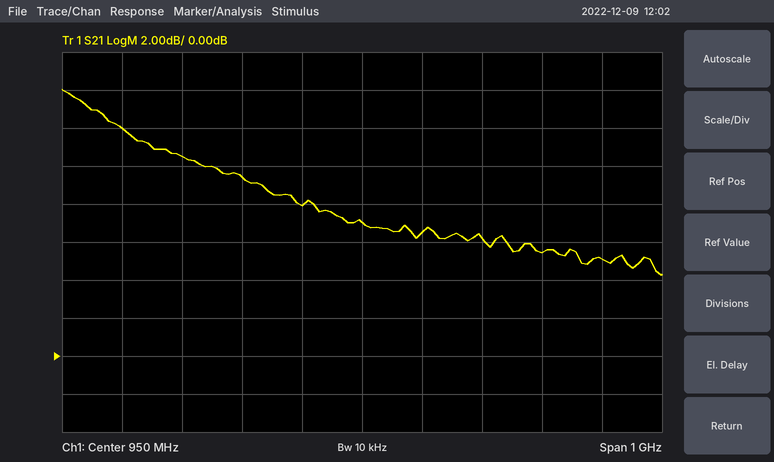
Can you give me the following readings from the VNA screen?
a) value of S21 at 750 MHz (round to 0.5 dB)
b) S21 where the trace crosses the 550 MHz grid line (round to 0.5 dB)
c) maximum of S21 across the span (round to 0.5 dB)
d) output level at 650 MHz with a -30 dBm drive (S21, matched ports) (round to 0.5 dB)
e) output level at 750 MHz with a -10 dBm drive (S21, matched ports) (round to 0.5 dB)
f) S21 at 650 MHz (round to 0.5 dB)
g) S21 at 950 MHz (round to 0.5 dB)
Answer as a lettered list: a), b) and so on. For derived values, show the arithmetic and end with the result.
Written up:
a) 9.5 dB
b) 12.0 dB
c) 14.0 dB
d) -30 dBm + (10.5 dB) = -19.5 dBm
e) -10 dBm + (9.5 dB) = -0.5 dBm
f) 10.5 dB
g) 7.0 dB
